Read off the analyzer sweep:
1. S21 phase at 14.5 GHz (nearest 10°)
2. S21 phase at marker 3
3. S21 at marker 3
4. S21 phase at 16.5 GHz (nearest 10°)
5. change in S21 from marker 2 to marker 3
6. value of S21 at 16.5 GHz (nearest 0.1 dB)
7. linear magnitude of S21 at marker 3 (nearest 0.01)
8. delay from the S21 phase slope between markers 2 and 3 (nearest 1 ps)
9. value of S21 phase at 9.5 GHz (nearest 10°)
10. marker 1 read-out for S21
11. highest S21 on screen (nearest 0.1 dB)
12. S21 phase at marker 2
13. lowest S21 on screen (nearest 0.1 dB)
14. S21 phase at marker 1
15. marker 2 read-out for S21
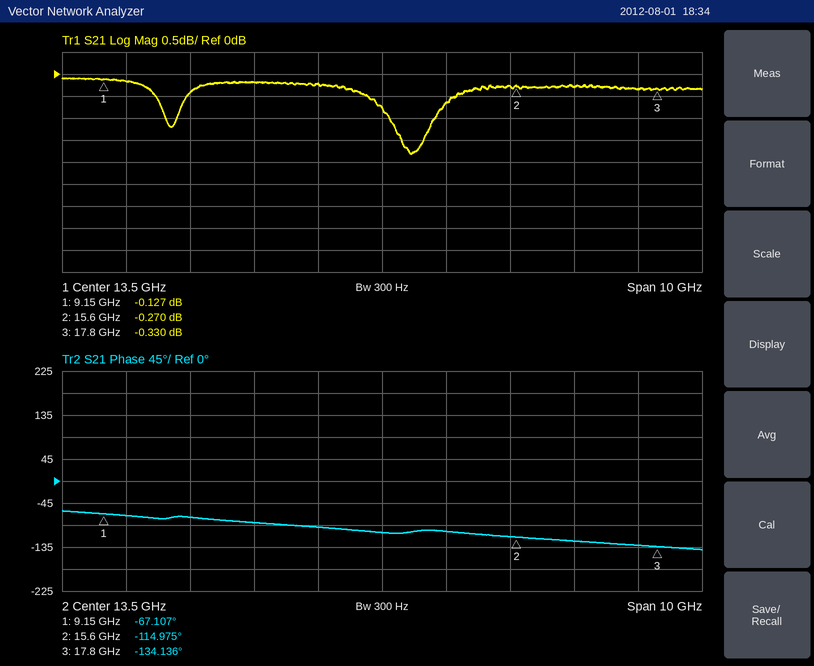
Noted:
-100°
-134.136°
-0.330 dB
-120°
-0.060 dB
-0.3 dB
0.96
24 ps
-70°
-0.127 dB
-0.1 dB
-114.975°
-1.8 dB
-67.107°
-0.270 dB
